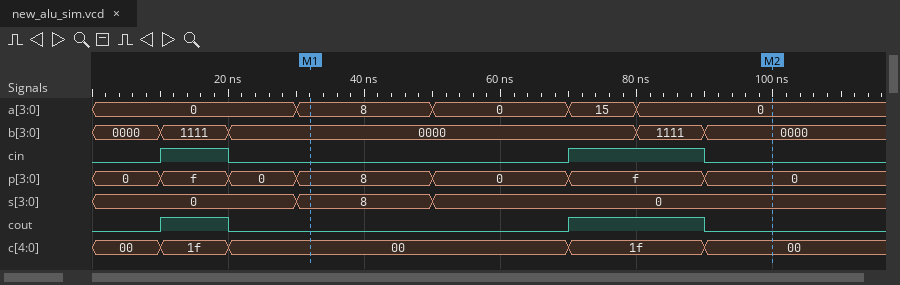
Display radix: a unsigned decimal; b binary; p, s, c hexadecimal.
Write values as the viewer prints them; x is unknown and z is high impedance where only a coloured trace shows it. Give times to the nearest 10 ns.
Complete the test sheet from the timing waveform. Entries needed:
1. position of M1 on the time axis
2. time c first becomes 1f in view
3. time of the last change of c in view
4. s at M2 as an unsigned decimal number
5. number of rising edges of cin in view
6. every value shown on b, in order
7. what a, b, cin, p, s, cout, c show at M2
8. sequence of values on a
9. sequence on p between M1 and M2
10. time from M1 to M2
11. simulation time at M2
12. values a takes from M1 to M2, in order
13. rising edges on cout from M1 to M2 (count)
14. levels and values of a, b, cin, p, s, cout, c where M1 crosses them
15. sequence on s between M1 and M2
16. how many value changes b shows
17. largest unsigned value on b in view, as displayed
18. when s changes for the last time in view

30 ns
10 ns
90 ns
0
2
0000, 1111, 0000, 1111, 0000
a=0, b=0000, cin=0, p=0, s=0, cout=0, c=00
0, 8, 0, 15, 0
8, 0, f, 0
70 ns
100 ns
8, 0, 15, 0
1
a=8, b=0000, cin=0, p=8, s=8, cout=0, c=00
8, 0
4
1111
50 ns
